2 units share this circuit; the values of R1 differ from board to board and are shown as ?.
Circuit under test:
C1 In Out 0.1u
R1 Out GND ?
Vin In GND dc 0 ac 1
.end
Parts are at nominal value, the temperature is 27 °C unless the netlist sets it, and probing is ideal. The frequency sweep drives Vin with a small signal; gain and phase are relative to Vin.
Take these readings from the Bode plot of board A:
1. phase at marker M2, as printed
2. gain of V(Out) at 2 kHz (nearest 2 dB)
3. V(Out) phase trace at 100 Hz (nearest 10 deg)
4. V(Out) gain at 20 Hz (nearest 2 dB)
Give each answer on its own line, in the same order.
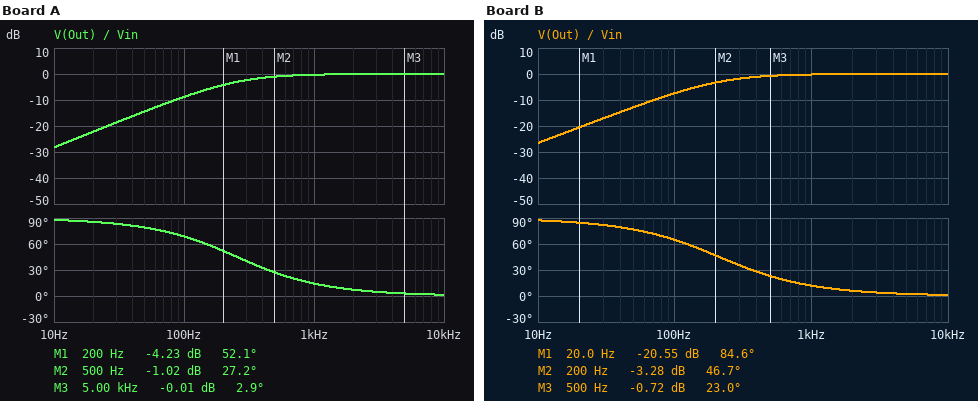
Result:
27.2 deg
0 dB
70 deg
-22 dB
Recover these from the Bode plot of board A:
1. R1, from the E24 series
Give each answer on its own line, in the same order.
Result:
6.2 kΩ
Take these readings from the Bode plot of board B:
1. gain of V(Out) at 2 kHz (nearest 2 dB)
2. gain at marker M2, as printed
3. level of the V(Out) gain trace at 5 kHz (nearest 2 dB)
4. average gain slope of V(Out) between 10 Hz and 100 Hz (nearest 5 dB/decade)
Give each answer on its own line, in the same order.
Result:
0 dB
-3.28 dB
0 dB
20 dB/decade
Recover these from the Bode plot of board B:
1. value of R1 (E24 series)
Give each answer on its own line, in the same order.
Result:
7.5 kΩ
